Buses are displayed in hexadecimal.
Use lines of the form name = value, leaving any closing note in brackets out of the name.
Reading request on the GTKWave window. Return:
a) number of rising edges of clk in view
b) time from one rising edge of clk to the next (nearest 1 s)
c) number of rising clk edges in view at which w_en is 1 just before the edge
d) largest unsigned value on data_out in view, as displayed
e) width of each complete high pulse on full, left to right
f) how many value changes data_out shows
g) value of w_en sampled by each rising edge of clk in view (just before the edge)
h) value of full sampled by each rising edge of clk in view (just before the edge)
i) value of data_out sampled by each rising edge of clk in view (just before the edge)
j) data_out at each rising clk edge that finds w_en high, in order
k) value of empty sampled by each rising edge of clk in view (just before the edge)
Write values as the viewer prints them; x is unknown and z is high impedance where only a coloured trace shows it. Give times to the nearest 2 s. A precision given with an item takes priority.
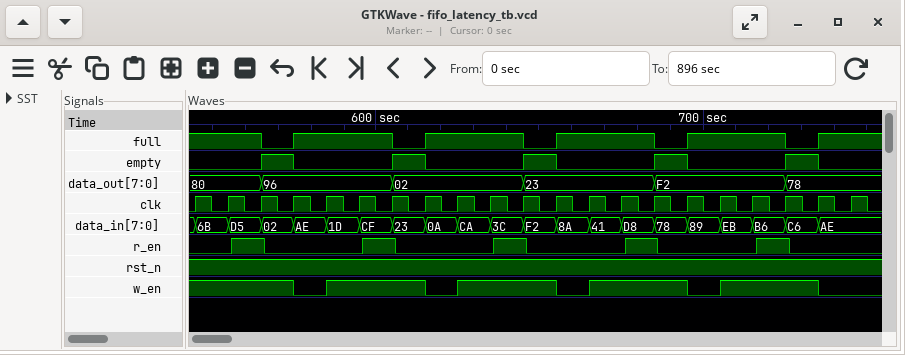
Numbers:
number of rising edges of clk in view = 21
time from one rising edge of clk to the next = 10 s
number of rising clk edges in view at which w_en is 1 just before the edge = 16
largest unsigned value on data_out in view, as displayed = F2
width of each complete high pulse on full, left to right = 30 s, 30 s, 30 s, 30 s
how many value changes data_out shows = 5
value of w_en sampled by each rising edge of clk in view = 1 1 1 1 0 1 1 1 0 1 1 1 0 1 1 1 0 1 1 1 0
value of full sampled by each rising edge of clk in view = 1 1 1 0 1 1 1 0 1 1 1 0 1 1 1 0 1 1 1 0 1
value of data_out sampled by each rising edge of clk in view = 80, 80, 80, 96, 96, 96, 96, 02, 02, 02, 02, 23, 23, 23, 23, F2, F2, F2, F2, 78, 78
data_out at each rising clk edge that finds w_en high, in order = 80, 80, 80, 96, 96, 96, 02, 02, 02, 23, 23, 23, F2, F2, F2, 78
value of empty sampled by each rising edge of clk in view = 0 0 0 1 0 0 0 1 0 0 0 1 0 0 0 1 0 0 0 1 0
